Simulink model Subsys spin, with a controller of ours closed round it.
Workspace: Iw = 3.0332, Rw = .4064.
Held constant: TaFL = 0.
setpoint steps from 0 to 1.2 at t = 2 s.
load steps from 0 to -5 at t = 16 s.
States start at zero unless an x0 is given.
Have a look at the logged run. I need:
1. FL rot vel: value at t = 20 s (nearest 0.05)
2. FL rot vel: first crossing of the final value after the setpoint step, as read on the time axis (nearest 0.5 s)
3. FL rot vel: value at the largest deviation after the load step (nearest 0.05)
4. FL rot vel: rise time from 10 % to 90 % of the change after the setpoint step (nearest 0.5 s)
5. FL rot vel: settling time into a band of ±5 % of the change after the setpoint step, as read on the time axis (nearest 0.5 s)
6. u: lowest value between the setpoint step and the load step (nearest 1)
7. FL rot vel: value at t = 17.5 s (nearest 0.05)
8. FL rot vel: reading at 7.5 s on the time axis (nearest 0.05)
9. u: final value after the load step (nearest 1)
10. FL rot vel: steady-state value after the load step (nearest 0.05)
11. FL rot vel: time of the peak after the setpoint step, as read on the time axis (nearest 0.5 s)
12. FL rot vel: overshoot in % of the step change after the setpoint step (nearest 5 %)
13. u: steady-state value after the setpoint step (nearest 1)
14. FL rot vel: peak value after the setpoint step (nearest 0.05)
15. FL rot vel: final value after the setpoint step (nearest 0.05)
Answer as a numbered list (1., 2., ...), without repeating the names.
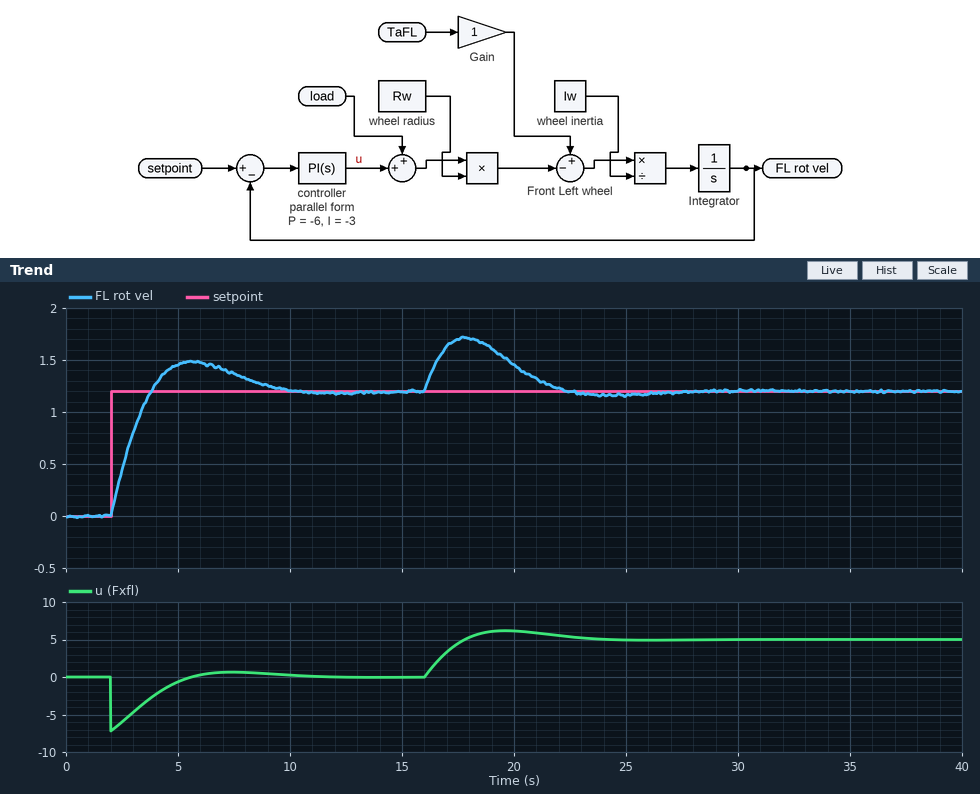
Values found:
1. 1.45
2. 4.0 s
3. 1.70
4. 1.5 s
5. 9.0 s
6. -7
7. 1.70
8. 1.35
9. 5
10. 1.20
11. 5.5 s
12. 25 %
13. 0
14. 1.50
15. 1.20
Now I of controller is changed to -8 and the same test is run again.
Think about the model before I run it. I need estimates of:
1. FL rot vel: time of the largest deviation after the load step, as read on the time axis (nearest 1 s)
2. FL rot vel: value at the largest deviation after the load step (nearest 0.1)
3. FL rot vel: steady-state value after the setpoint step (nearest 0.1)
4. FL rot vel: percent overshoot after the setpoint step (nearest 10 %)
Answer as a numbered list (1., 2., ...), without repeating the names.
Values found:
1. 17 s
2. 1.6
3. 1.2
4. 40 %
